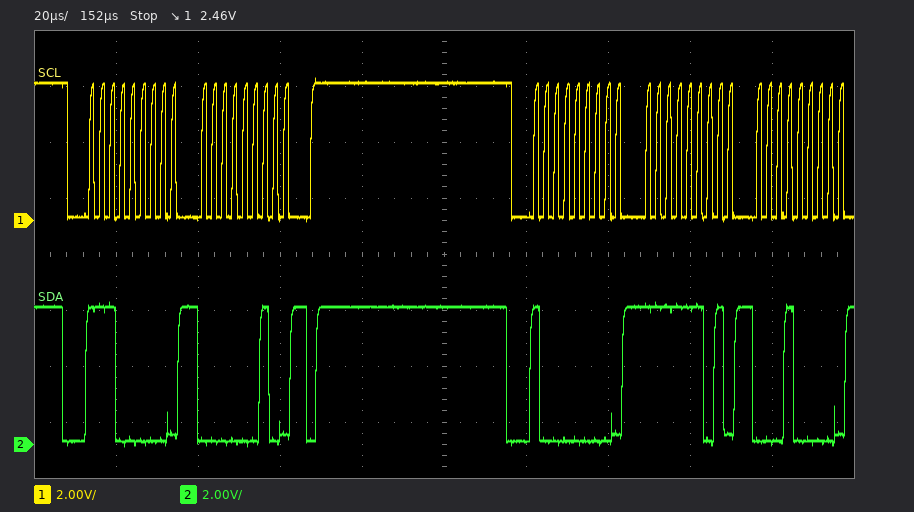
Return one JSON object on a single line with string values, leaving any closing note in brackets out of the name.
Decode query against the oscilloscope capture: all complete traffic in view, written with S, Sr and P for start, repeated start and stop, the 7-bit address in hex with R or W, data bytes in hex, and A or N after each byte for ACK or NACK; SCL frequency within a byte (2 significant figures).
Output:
{"all complete traffic in view, written with S, Sr and P for start, repeated start and stop, the 7-bit address in hex with R or W, data bytes in hex, and A or N after each byte for ACK or NACK": "S 70W A 02 A P S 40W A FD A 10 A", "SCL frequency within a byte": "400 kHz"}
